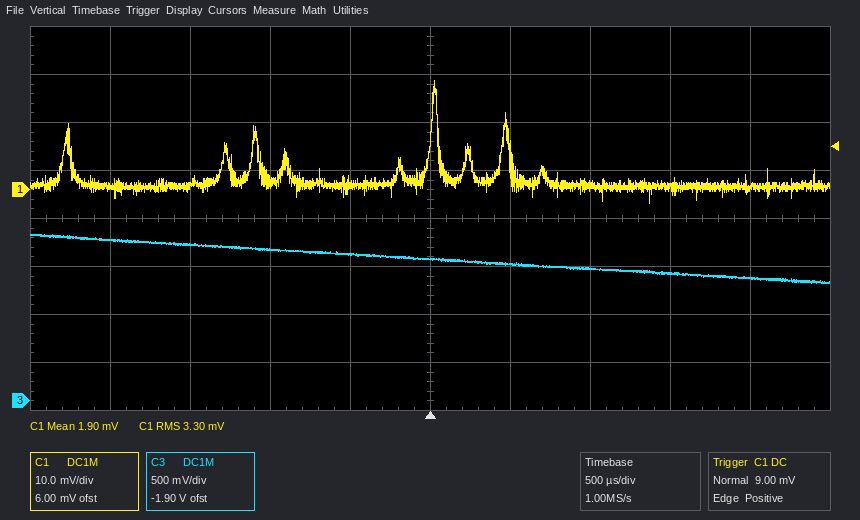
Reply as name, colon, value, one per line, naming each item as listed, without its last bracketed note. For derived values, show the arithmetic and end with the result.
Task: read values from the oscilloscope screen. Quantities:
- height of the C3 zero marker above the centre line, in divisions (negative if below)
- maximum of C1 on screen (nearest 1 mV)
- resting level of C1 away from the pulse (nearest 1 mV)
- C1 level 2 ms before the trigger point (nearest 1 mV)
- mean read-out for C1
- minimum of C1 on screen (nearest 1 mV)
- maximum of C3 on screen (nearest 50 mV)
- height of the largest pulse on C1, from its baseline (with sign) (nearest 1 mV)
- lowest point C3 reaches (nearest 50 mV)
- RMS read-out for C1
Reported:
height of the C3 zero marker above the centre line, in divisions: -3.8 div
maximum of C1 on screen: 23 mV
resting level of C1 away from the pulse: 1 mV
C1 level 2 ms before the trigger point: 1 mV
mean read-out for C1: 1.90 mV
minimum of C1 on screen: -3 mV
maximum of C3 on screen: 1.75 V
height of the largest pulse on C1, from its baseline (with sign): 23 mV − (1 mV) = +22 mV
lowest point C3 reaches: 1.20 V
RMS read-out for C1: 3.30 mV
